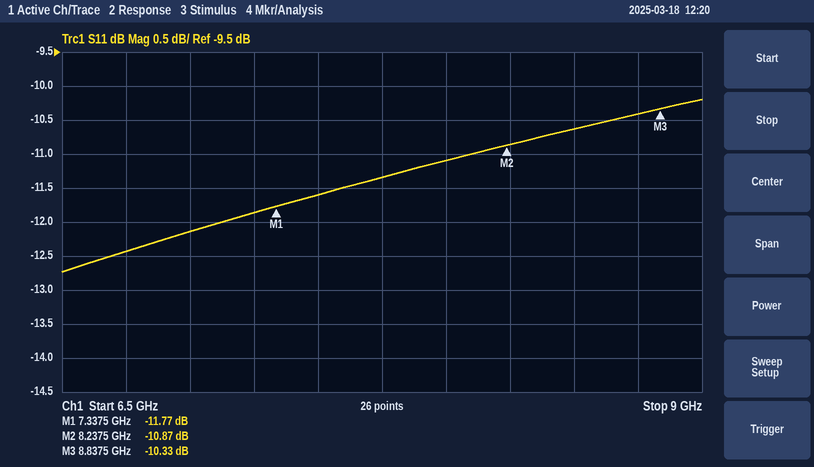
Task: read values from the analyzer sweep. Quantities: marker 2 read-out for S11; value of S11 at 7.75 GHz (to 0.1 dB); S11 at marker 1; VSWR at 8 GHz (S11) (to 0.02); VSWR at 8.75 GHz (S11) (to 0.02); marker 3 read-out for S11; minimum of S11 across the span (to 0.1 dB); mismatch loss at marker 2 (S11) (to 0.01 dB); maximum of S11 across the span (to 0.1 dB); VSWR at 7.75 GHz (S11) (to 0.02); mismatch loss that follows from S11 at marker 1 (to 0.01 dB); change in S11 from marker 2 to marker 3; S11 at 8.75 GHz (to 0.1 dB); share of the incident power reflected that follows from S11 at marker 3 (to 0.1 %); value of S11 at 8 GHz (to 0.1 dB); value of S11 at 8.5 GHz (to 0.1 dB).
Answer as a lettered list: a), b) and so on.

a) -10.87 dB
b) -11.3 dB
c) -11.77 dB
d) 1.78
e) 1.86
f) -10.33 dB
g) -12.7 dB
h) 0.37 dB
i) -10.2 dB
j) 1.74
k) 0.30 dB
l) 0.54 dB
m) -10.4 dB
n) 9.3 %
o) -11.1 dB
p) -10.6 dB
